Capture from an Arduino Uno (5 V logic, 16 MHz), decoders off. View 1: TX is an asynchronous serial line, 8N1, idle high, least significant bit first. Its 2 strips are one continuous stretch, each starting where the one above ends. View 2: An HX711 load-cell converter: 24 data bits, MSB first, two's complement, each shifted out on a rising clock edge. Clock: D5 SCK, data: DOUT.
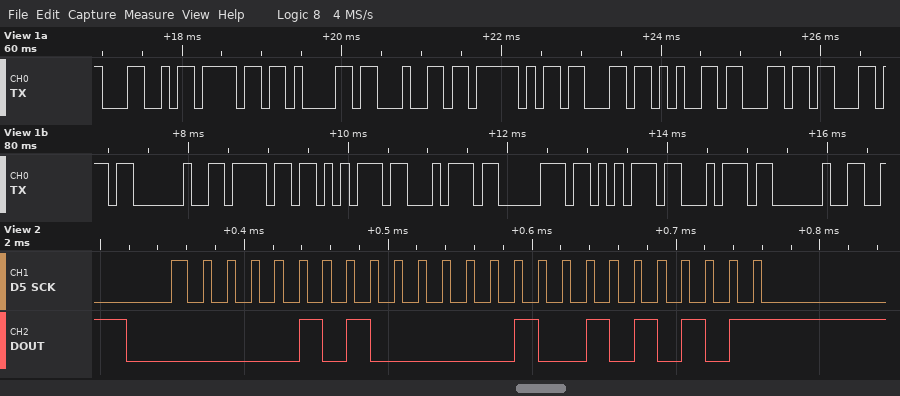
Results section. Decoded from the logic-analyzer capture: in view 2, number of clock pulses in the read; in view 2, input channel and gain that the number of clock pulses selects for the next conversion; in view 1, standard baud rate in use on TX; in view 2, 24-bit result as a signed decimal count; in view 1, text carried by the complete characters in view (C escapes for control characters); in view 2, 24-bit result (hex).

25
channel A, gain 128
9600 baud
328277
"Load_cell output "
0x050255
